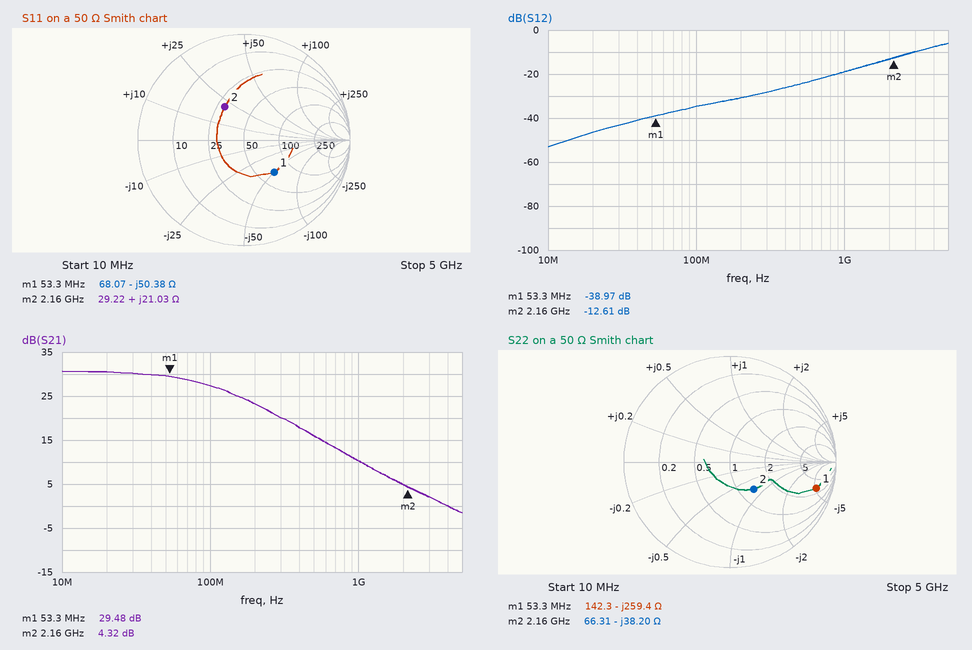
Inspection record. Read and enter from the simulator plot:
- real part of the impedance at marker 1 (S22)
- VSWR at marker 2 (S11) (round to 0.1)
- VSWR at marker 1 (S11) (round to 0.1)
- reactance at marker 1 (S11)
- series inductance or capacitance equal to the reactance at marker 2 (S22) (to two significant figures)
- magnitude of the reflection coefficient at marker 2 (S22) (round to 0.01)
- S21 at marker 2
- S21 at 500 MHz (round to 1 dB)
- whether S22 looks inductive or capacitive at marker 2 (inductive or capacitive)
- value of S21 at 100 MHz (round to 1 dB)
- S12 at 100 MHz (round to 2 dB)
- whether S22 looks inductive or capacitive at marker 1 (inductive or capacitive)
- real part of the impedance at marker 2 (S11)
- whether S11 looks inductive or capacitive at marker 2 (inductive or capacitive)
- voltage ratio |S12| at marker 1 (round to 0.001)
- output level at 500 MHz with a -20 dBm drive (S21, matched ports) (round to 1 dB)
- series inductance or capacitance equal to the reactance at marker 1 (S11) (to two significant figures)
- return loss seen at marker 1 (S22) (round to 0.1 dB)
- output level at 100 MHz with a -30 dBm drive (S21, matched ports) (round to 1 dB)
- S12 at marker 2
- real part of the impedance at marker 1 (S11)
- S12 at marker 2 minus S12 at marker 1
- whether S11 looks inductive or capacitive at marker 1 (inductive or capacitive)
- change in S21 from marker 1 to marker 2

142.3 Ω
2.1
2.4
-50.38 Ω
1.9 pF
0.34
4.32 dB
16 dB
capacitive
27 dB
-34 dB
capacitive
29.22 Ω
inductive
0.011
-4 dBm
59 pF
1.4 dB
-3 dBm
-12.61 dB
68.07 Ω
26.36 dB
capacitive
-25.16 dB
